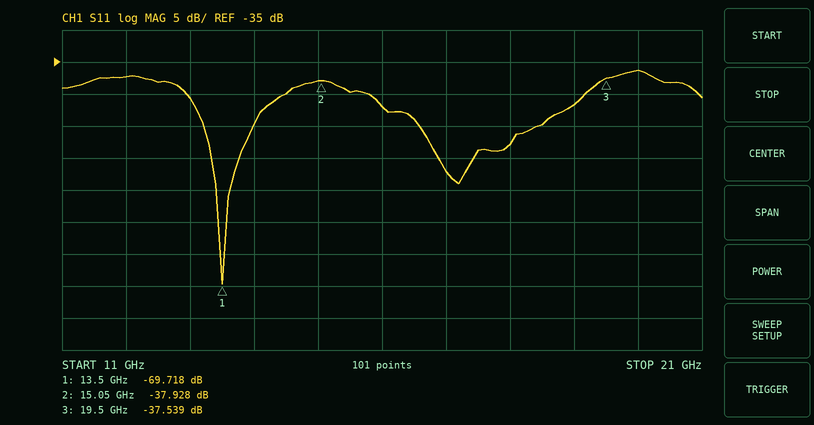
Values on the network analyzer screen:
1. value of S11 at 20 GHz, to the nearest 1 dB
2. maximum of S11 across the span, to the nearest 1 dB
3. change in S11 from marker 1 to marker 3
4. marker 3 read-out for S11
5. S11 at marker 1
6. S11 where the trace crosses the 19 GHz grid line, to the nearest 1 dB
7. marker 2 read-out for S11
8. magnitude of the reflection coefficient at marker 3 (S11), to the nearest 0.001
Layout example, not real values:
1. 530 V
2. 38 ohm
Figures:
1. -36 dB
2. -36 dB
3. 32.179 dB
4. -37.539 dB
5. -69.718 dB
6. -42 dB
7. -37.928 dB
8. 0.013
